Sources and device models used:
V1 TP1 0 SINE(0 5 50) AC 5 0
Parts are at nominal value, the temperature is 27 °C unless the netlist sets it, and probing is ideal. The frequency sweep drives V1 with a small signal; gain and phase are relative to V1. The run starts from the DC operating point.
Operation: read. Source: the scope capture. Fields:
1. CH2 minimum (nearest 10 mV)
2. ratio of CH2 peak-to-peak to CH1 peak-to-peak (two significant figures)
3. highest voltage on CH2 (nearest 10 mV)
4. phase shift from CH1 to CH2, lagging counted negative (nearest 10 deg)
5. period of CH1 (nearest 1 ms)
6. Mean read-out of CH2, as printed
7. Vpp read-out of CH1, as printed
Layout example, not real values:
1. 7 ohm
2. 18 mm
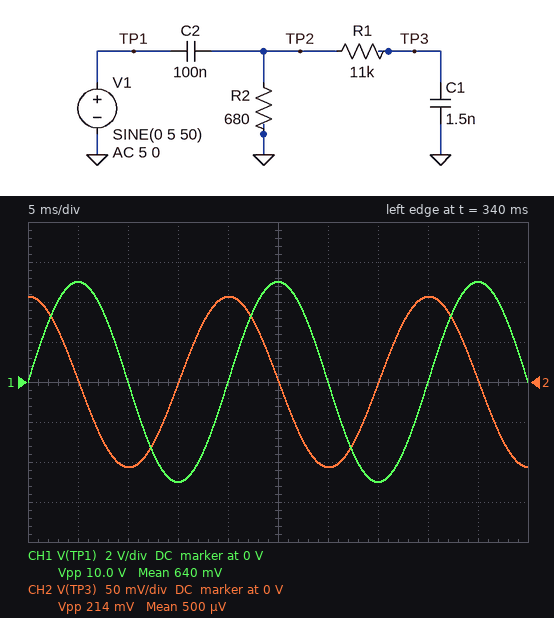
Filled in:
1. -110 mV
2. 0.021
3. 110 mV
4. 90 deg
5. 20 ms
6. 500 µV
7. 10.0 V
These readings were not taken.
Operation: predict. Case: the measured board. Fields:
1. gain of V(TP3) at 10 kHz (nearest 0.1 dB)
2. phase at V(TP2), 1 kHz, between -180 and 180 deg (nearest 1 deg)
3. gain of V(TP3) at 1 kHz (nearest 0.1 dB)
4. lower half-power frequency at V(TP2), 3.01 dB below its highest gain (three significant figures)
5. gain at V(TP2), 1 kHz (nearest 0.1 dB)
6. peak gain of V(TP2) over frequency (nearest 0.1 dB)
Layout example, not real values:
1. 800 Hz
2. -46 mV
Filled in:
1. -3.5 dB
2. 67 deg
3. -8.2 dB
4. 2.38 kHz
5. -8.1 dB
6. 0 dB
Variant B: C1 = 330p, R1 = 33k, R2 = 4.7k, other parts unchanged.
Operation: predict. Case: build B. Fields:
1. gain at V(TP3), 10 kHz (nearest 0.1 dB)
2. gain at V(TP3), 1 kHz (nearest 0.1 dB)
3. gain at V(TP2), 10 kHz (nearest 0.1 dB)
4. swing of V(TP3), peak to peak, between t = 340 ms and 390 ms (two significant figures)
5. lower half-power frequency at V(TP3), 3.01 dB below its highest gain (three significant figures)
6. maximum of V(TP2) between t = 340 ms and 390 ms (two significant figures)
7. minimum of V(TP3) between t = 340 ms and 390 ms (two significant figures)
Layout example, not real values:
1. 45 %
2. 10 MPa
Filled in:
1. -1.7 dB
2. -0.5 dB
3. 0 dB
4. 1.5 V
5. 323 Hz
6. 730 mV
7. -730 mV
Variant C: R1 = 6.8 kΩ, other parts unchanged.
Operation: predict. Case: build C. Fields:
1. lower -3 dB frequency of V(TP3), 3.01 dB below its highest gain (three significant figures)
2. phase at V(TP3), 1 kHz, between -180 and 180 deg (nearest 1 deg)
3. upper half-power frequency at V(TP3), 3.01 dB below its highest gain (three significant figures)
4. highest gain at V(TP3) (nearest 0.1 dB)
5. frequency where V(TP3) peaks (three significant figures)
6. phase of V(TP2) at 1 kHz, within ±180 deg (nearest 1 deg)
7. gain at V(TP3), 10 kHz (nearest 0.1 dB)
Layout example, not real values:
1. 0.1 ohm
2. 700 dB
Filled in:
1. 1.83 kHz
2. 63 deg
3. 20.0 kHz
4. -1.3 dB
5. 6.04 kHz
6. 67 deg
7. -1.8 dB
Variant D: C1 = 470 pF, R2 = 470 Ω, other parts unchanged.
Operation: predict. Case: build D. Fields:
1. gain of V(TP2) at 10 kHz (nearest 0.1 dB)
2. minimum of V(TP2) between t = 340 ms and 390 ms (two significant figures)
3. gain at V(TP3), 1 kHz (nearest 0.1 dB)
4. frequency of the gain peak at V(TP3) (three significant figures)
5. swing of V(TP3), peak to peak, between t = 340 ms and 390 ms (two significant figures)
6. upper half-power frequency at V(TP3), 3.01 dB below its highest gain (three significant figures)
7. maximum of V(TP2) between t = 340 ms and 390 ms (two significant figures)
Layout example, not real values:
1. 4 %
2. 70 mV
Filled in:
1. -0.5 dB
2. -74 mV
3. -11.0 dB
4. 10.2 kHz
5. 150 mV
6. 37.1 kHz
7. 74 mV
